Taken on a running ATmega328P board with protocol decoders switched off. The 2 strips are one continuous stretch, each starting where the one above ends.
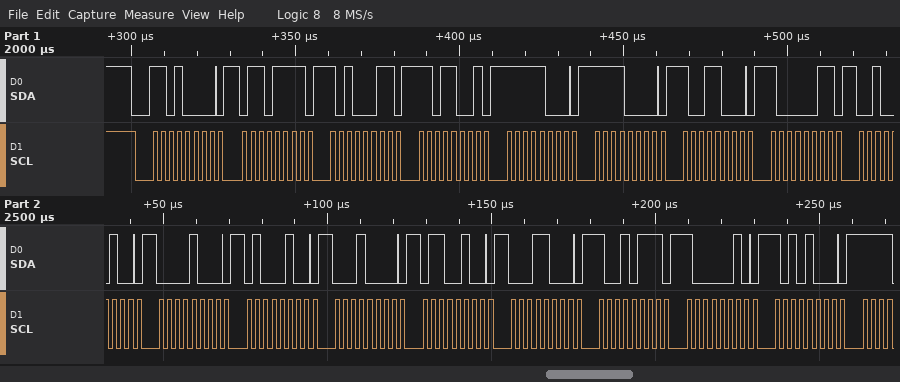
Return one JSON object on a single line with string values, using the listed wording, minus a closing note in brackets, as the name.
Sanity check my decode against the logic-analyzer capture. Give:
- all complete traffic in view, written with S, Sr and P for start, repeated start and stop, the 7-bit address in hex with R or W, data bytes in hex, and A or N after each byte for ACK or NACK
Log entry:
{"all complete traffic in view, written with S, Sr and P for start, repeated start and stop, the 7-bit address in hex with R or W, data bytes in hex, and A or N after each byte for ACK or NACK": "S 68W A 6F A A3 A D9 A F8 A F0 A 98 A 83 A 24 A 08 A 44 A 10 A 64 A 18 A 97 A 82 A A8 A"}
